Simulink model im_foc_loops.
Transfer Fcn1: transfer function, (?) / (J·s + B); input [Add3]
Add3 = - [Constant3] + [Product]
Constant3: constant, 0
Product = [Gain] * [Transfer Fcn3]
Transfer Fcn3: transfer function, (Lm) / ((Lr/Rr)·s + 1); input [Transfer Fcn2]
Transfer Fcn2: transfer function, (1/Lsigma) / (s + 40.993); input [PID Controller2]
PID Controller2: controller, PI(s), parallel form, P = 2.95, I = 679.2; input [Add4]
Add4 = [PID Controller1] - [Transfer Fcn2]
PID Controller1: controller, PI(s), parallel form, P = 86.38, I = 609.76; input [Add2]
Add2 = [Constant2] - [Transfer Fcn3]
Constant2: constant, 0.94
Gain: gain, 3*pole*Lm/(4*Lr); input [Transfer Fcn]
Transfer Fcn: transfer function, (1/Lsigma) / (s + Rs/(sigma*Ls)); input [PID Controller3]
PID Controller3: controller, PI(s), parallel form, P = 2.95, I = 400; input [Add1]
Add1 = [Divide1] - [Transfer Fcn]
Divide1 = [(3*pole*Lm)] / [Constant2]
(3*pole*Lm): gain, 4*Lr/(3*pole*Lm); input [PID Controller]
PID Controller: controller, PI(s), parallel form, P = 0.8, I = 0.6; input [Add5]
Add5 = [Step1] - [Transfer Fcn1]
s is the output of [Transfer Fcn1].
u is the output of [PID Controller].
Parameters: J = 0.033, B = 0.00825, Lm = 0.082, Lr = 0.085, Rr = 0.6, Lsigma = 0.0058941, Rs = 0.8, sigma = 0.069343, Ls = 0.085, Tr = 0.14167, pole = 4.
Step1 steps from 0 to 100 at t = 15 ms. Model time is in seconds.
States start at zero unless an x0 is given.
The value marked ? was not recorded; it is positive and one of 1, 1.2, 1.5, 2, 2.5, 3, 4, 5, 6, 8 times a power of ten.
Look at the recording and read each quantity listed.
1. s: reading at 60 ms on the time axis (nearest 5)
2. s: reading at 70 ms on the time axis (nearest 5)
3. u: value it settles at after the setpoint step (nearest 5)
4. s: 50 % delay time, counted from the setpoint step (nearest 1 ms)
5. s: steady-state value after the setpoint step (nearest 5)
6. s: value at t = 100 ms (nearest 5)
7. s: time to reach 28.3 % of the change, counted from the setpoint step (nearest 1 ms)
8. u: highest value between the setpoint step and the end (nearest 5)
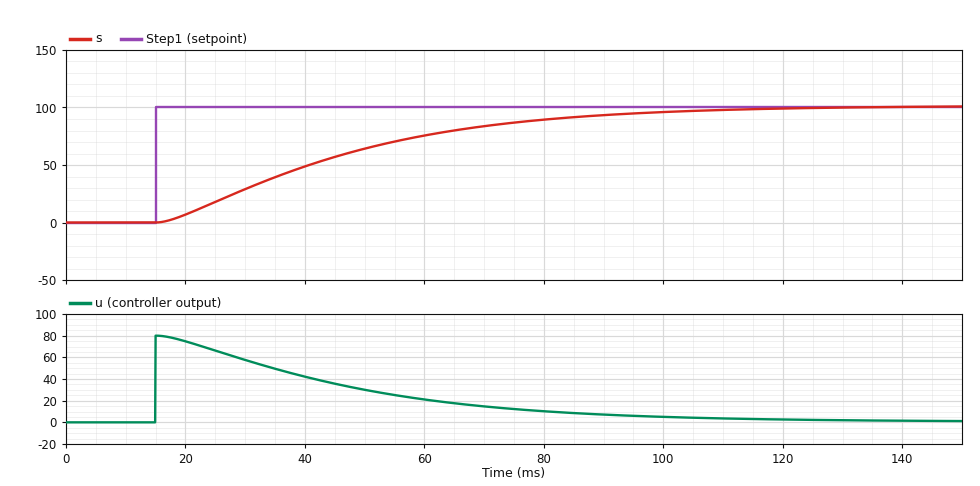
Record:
75
85
0
26 ms
100
95
15 ms
80
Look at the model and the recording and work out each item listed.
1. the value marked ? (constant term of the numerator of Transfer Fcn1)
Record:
1.5
